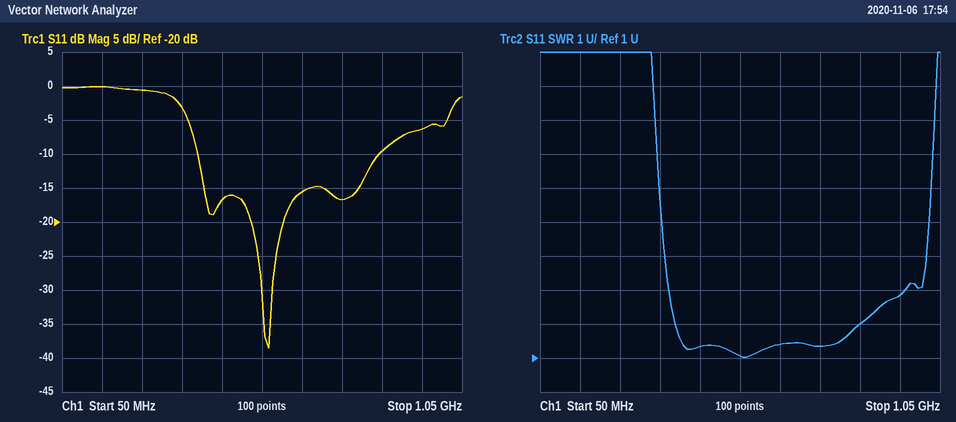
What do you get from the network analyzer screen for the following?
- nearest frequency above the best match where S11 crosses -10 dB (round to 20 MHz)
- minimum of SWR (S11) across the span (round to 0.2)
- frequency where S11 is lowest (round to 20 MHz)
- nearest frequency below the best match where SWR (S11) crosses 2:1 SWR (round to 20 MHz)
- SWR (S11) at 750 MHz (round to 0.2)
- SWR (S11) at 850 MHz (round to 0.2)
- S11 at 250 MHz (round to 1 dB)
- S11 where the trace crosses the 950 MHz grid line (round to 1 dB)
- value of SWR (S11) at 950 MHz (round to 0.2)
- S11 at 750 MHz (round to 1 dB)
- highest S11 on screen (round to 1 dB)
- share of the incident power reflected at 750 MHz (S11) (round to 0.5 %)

840 MHz
1.0
560 MHz
380 MHz
1.4
2.0
-1 dB
-6 dB
2.8
-17 dB
0 dB
2.0 %
